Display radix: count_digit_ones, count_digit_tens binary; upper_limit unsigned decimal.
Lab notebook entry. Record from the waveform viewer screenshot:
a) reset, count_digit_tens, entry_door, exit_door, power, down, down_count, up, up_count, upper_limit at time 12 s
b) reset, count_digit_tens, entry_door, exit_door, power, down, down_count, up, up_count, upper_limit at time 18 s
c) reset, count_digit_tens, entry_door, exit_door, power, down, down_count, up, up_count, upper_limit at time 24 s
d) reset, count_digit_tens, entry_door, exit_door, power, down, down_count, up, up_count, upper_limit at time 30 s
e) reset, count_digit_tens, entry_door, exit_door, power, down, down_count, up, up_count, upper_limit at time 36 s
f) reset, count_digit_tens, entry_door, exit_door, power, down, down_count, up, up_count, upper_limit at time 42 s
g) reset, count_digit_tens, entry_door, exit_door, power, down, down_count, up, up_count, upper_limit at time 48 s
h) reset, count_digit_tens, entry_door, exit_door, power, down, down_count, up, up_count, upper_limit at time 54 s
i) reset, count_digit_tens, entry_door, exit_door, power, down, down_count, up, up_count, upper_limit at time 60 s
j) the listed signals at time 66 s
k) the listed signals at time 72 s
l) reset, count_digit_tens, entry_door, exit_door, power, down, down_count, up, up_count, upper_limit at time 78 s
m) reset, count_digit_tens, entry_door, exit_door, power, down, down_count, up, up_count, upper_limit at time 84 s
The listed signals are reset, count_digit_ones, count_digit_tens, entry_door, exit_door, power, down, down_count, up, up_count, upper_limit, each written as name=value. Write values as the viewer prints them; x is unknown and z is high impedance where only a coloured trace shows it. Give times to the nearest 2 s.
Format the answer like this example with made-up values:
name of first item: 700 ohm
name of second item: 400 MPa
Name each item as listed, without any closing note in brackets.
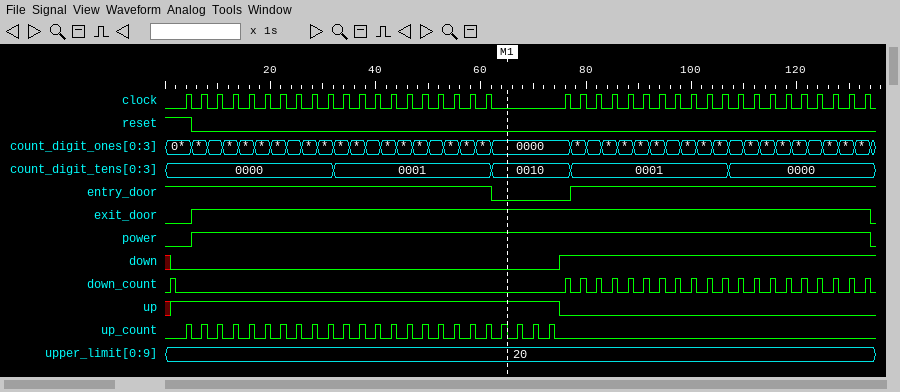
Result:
reset, count_digit_tens, entry_door, exit_door, power, down, down_count, up, up_count, upper_limit at time 12 s: reset=0, count_digit_tens=0000, entry_door=1, exit_door=1, power=1, down=0, down_count=0, up=1, up_count=0, upper_limit=20
reset, count_digit_tens, entry_door, exit_door, power, down, down_count, up, up_count, upper_limit at time 18 s: reset=0, count_digit_tens=0000, entry_door=1, exit_door=1, power=1, down=0, down_count=0, up=1, up_count=0, upper_limit=20
reset, count_digit_tens, entry_door, exit_door, power, down, down_count, up, up_count, upper_limit at time 24 s: reset=0, count_digit_tens=0000, entry_door=1, exit_door=1, power=1, down=0, down_count=0, up=1, up_count=0, upper_limit=20
reset, count_digit_tens, entry_door, exit_door, power, down, down_count, up, up_count, upper_limit at time 30 s: reset=0, count_digit_tens=0000, entry_door=1, exit_door=1, power=1, down=0, down_count=0, up=1, up_count=0, upper_limit=20
reset, count_digit_tens, entry_door, exit_door, power, down, down_count, up, up_count, upper_limit at time 36 s: reset=0, count_digit_tens=0001, entry_door=1, exit_door=1, power=1, down=0, down_count=0, up=1, up_count=0, upper_limit=20
reset, count_digit_tens, entry_door, exit_door, power, down, down_count, up, up_count, upper_limit at time 42 s: reset=0, count_digit_tens=0001, entry_door=1, exit_door=1, power=1, down=0, down_count=0, up=1, up_count=0, upper_limit=20
reset, count_digit_tens, entry_door, exit_door, power, down, down_count, up, up_count, upper_limit at time 48 s: reset=0, count_digit_tens=0001, entry_door=1, exit_door=1, power=1, down=0, down_count=0, up=1, up_count=0, upper_limit=20
reset, count_digit_tens, entry_door, exit_door, power, down, down_count, up, up_count, upper_limit at time 54 s: reset=0, count_digit_tens=0001, entry_door=1, exit_door=1, power=1, down=0, down_count=0, up=1, up_count=0, upper_limit=20
reset, count_digit_tens, entry_door, exit_door, power, down, down_count, up, up_count, upper_limit at time 60 s: reset=0, count_digit_tens=0001, entry_door=1, exit_door=1, power=1, down=0, down_count=0, up=1, up_count=0, upper_limit=20
the listed signals at time 66 s: reset=0, count_digit_ones=0000, count_digit_tens=0010, entry_door=0, exit_door=1, power=1, down=0, down_count=0, up=1, up_count=0, upper_limit=20
the listed signals at time 72 s: reset=0, count_digit_ones=0000, count_digit_tens=0010, entry_door=0, exit_door=1, power=1, down=0, down_count=0, up=1, up_count=0, upper_limit=20
reset, count_digit_tens, entry_door, exit_door, power, down, down_count, up, up_count, upper_limit at time 78 s: reset=0, count_digit_tens=0001, entry_door=1, exit_door=1, power=1, down=1, down_count=0, up=0, up_count=0, upper_limit=20
reset, count_digit_tens, entry_door, exit_door, power, down, down_count, up, up_count, upper_limit at time 84 s: reset=0, count_digit_tens=0001, entry_door=1, exit_door=1, power=1, down=1, down_count=0, up=0, up_count=0, upper_limit=20
